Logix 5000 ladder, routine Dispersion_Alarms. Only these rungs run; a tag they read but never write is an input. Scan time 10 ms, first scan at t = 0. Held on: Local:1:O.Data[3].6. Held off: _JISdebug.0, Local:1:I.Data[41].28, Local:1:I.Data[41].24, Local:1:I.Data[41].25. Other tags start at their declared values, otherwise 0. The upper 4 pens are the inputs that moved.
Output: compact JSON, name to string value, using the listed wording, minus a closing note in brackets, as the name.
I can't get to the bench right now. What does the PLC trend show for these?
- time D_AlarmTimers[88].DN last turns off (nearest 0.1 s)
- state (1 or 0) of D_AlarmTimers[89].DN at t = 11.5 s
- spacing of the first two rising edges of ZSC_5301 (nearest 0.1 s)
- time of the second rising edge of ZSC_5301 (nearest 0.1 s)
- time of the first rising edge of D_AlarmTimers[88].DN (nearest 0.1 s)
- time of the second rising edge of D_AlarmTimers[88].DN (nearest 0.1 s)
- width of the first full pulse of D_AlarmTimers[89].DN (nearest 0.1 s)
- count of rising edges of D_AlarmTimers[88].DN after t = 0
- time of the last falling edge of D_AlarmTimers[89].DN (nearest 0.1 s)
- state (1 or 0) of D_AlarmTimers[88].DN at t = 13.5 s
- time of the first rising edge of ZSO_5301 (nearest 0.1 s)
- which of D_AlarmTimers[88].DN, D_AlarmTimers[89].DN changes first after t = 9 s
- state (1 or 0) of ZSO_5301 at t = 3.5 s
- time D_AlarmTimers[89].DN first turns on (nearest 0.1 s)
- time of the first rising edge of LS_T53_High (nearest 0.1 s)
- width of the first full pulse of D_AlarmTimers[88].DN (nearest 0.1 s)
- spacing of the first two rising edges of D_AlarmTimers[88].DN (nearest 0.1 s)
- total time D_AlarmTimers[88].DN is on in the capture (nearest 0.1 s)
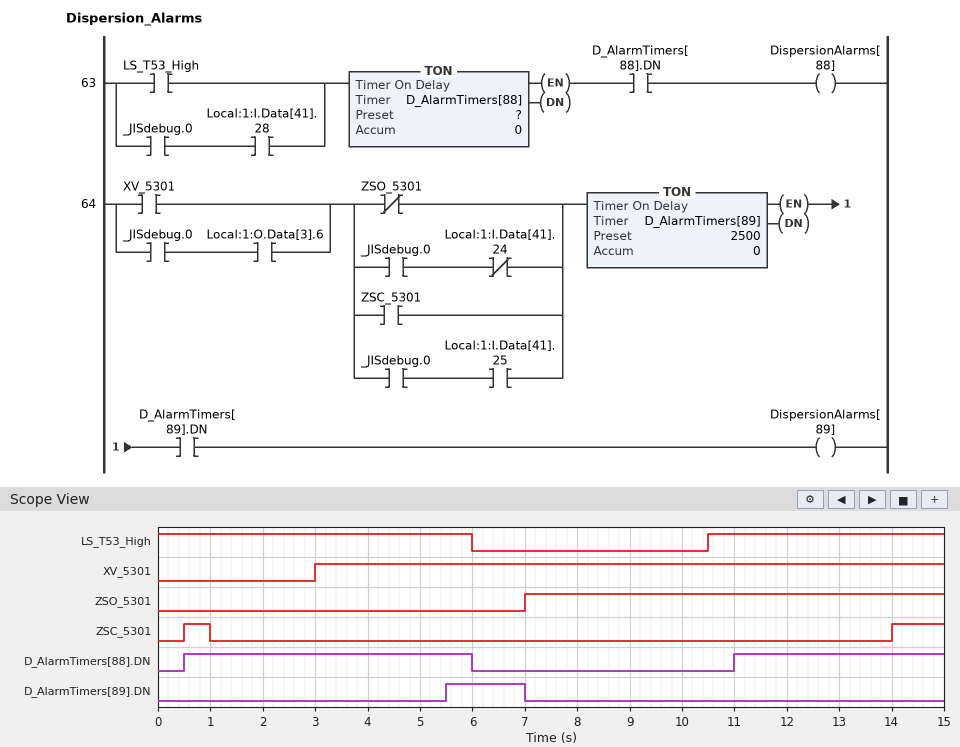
{"time D_AlarmTimers[88].DN last turns off": "6.0 s", "state (1 or 0) of D_AlarmTimers[89].DN at t = 11.5 s": "0", "spacing of the first two rising edges of ZSC_5301": "13.5 s", "time of the second rising edge of ZSC_5301": "14.0 s", "time of the first rising edge of D_AlarmTimers[88].DN": "0.5 s", "time of the second rising edge of D_AlarmTimers[88].DN": "11.0 s", "width of the first full pulse of D_AlarmTimers[89].DN": "1.5 s", "count of rising edges of D_AlarmTimers[88].DN after t = 0": "2", "time of the last falling edge of D_AlarmTimers[89].DN": "7.0 s", "state (1 or 0) of D_AlarmTimers[88].DN at t = 13.5 s": "1", "time of the first rising edge of ZSO_5301": "7.0 s", "which of D_AlarmTimers[88].DN, D_AlarmTimers[89].DN changes first after t = 9 s": "D_AlarmTimers[88].DN", "state (1 or 0) of ZSO_5301 at t = 3.5 s": "0", "time D_AlarmTimers[89].DN first turns on": "5.5 s", "time of the first rising edge of LS_T53_High": "10.5 s", "width of the first full pulse of D_AlarmTimers[88].DN": "5.5 s", "spacing of the first two rising edges of D_AlarmTimers[88].DN": "10.5 s", "total time D_AlarmTimers[88].DN is on in the capture": "9.5 s"}
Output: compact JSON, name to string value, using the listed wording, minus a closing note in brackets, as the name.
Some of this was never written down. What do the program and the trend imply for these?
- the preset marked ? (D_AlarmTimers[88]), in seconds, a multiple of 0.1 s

{"the preset marked ? (D_AlarmTimers[88]), in seconds, a multiple of 0.1 s": "0.5 s"}
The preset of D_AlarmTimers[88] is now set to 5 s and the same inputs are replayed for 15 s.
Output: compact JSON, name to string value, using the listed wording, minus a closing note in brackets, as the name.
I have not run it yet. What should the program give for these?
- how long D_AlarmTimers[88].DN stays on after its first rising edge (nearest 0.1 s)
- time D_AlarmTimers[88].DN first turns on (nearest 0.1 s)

{"how long D_AlarmTimers[88].DN stays on after its first rising edge": "1.0 s", "time D_AlarmTimers[88].DN first turns on": "5.0 s"}
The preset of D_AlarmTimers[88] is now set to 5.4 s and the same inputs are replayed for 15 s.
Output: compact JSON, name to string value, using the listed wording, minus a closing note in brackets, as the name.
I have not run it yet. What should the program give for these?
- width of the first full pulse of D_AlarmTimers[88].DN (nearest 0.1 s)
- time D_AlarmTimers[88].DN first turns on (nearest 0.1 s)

{"width of the first full pulse of D_AlarmTimers[88].DN": "0.6 s", "time D_AlarmTimers[88].DN first turns on": "5.4 s"}
